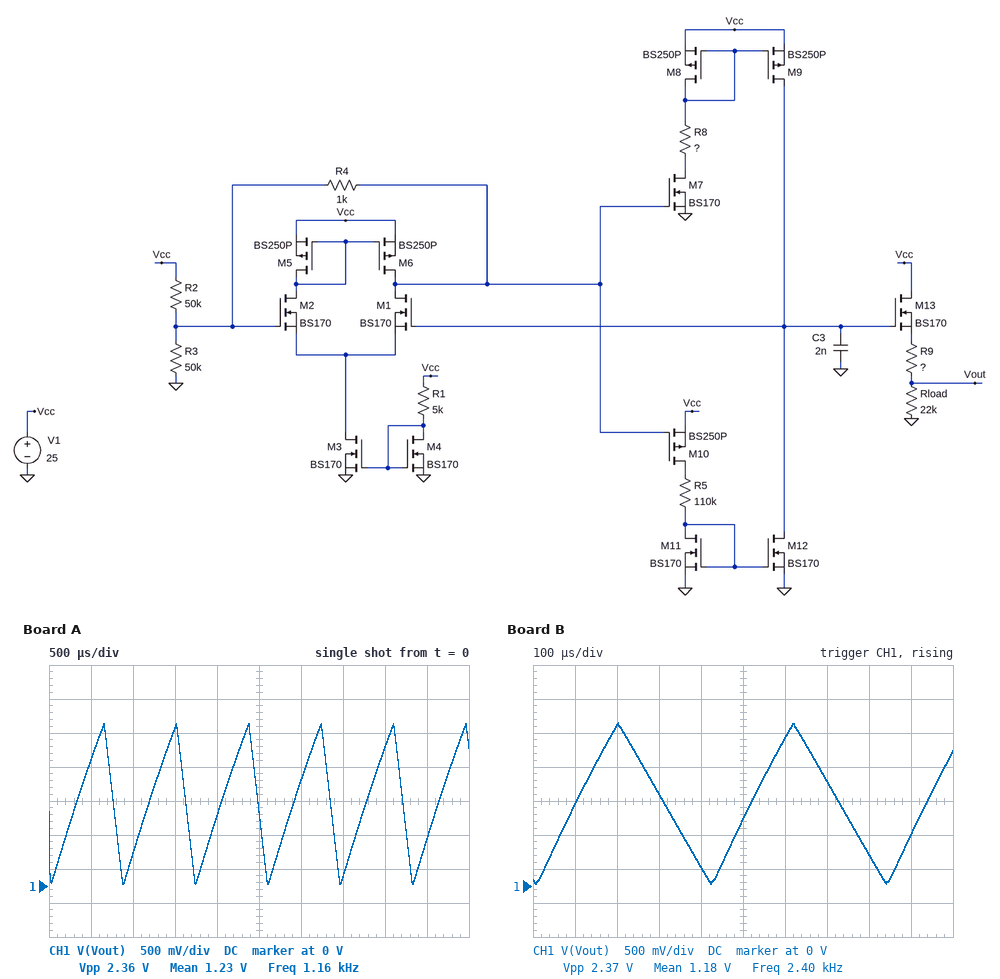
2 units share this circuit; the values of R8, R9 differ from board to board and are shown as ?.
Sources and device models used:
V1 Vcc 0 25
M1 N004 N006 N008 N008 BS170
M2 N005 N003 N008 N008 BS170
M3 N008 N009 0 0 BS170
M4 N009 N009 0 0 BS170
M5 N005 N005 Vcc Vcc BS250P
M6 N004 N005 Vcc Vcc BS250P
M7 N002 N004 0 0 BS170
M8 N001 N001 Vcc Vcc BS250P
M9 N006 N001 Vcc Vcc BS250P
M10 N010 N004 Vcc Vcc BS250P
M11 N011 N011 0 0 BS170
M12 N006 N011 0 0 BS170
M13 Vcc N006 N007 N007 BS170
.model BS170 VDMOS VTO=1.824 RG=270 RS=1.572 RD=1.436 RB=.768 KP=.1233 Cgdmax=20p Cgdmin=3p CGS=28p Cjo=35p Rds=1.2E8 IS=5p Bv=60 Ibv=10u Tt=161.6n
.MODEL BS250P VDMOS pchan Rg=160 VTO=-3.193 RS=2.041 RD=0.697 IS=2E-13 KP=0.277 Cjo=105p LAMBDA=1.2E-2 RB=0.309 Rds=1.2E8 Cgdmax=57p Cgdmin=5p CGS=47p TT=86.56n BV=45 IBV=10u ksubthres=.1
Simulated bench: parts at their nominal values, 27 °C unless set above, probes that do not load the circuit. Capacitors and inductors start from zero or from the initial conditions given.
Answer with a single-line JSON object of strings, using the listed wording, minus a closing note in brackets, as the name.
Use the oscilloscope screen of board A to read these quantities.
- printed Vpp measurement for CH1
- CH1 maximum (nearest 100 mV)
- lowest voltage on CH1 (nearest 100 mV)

{"printed Vpp measurement for CH1": "2.36 V", "CH1 maximum": "2.4 V", "lowest voltage on CH1": "0 V"}
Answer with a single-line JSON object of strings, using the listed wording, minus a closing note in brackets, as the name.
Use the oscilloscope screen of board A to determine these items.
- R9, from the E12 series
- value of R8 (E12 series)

{"R9, from the E12 series": "180 kΩ", "value of R8": "330 kΩ"}
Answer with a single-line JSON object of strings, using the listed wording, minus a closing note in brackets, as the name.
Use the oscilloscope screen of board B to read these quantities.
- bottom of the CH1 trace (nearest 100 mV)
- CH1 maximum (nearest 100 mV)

{"bottom of the CH1 trace": "0 V", "CH1 maximum": "2.4 V"}
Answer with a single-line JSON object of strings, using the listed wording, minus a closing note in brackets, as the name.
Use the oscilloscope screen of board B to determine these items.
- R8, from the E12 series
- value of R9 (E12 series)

{"R8, from the E12 series": "100 kΩ", "value of R9": "180 kΩ"}
